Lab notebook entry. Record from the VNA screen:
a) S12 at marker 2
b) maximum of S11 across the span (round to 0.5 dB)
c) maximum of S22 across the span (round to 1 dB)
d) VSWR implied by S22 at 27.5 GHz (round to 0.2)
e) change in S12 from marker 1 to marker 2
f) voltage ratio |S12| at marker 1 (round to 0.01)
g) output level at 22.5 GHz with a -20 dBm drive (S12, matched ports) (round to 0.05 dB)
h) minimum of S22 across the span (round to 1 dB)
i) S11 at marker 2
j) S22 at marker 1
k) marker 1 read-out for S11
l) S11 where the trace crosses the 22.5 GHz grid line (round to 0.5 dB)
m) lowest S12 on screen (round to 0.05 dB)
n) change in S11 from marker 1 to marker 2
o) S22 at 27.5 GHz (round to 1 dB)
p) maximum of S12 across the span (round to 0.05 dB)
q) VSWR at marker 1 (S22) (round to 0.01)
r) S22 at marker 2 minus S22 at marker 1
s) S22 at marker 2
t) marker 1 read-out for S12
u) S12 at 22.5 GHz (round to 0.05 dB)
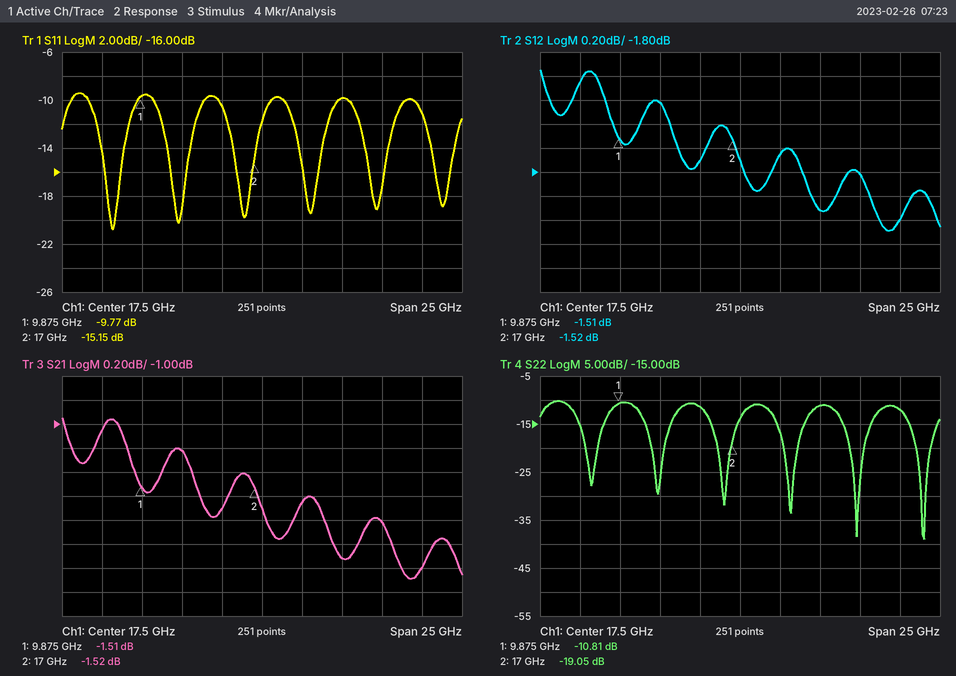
-1.52 dB
-9.5 dB
-10 dB
1.6
-0.01 dB
0.84
-22.10 dBm
-39 dB
-15.15 dB
-10.81 dB
-9.77 dB
-10.0 dB
-2.30 dB
-5.38 dB
-12 dB
-0.95 dB
1.81
-8.24 dB
-19.05 dB
-1.51 dB
-2.10 dB
